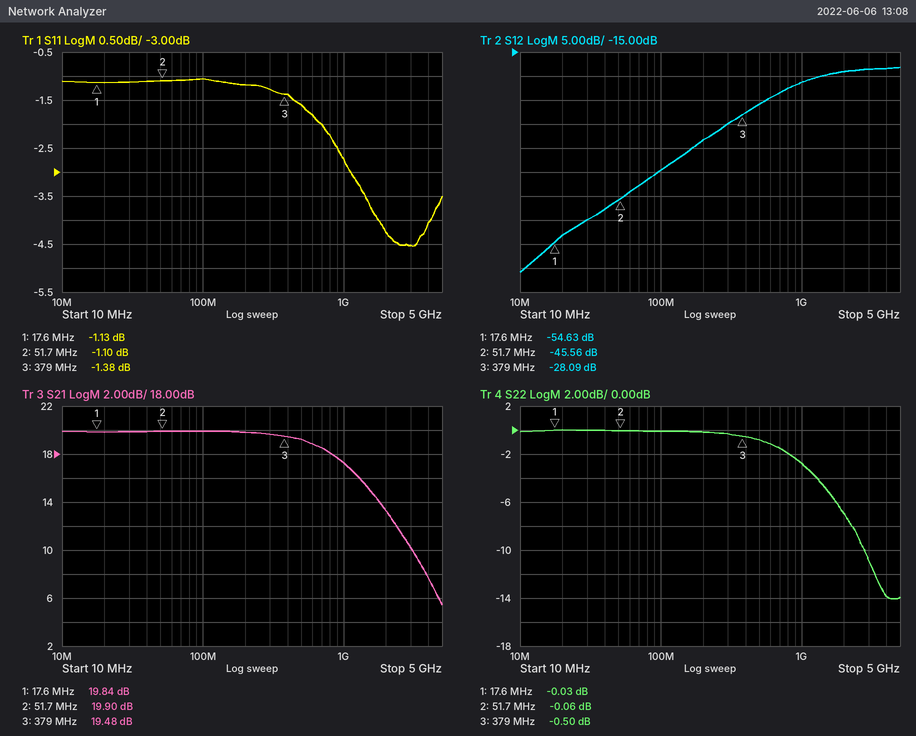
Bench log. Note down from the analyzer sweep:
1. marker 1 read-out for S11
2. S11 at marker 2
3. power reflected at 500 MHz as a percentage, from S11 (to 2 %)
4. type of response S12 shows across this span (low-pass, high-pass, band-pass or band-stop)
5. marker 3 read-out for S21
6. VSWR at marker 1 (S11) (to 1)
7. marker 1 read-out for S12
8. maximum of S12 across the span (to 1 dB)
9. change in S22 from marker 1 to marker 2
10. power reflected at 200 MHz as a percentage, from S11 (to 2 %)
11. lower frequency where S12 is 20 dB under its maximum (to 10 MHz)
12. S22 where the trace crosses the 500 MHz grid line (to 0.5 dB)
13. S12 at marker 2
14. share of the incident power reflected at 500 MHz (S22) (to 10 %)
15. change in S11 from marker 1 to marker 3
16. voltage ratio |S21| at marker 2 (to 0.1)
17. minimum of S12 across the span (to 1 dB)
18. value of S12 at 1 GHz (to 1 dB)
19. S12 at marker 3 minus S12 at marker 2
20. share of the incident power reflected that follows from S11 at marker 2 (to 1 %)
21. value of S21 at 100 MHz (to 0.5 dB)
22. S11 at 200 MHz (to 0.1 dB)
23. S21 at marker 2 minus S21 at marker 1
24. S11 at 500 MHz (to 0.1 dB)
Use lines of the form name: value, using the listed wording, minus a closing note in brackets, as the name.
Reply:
marker 1 read-out for S11: -1.13 dB
S11 at marker 2: -1.10 dB
power reflected at 500 MHz as a percentage, from S11: 70 %
type of response S12 shows across this span: high-pass
marker 3 read-out for S21: 19.48 dB
VSWR at marker 1 (S11): 15
marker 1 read-out for S12: -54.63 dB
maximum of S12 across the span: -18 dB
change in S22 from marker 1 to marker 2: -0.03 dB
power reflected at 200 MHz as a percentage, from S11: 76 %
lower frequency where S12 is 20 dB under its maximum: 120 MHz
S22 where the trace crosses the 500 MHz grid line: -1.0 dB
S12 at marker 2: -45.56 dB
share of the incident power reflected at 500 MHz (S22): 80 %
change in S11 from marker 1 to marker 3: -0.25 dB
voltage ratio |S21| at marker 2: 9.9
minimum of S12 across the span: -61 dB
value of S12 at 1 GHz: -21 dB
S12 at marker 3 minus S12 at marker 2: 17.47 dB
share of the incident power reflected that follows from S11 at marker 2: 78 %
value of S21 at 100 MHz: 20.0 dB
S11 at 200 MHz: -1.2 dB
S21 at marker 2 minus S21 at marker 1: 0.06 dB
S11 at 500 MHz: -1.6 dB
